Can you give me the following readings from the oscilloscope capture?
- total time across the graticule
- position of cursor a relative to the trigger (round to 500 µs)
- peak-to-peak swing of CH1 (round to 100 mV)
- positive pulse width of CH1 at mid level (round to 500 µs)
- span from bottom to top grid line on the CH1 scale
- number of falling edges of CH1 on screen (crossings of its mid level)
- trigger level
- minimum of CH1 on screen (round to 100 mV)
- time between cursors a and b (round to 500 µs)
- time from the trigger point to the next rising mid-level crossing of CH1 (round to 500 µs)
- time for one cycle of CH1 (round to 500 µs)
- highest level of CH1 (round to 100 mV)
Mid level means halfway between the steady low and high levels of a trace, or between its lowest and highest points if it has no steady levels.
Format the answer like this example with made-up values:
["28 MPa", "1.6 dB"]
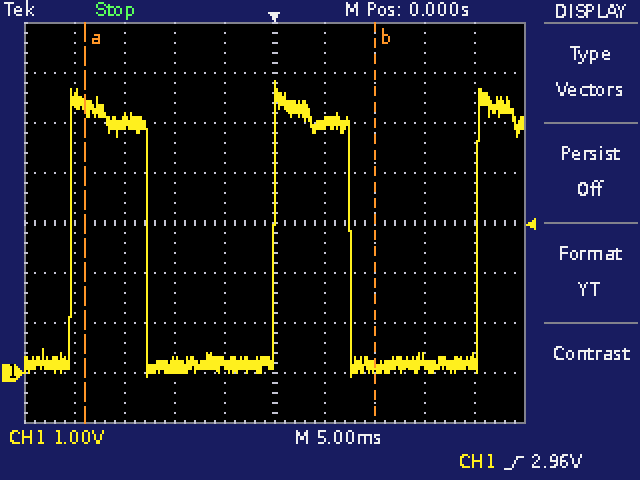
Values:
["50 ms", "-19.0 ms", "5.9 V", "7.5 ms", "8 V", "2", "2.96 V", "-100 mV", "29.0 ms", "20.5 ms", "20.5 ms", "5.8 V"]
